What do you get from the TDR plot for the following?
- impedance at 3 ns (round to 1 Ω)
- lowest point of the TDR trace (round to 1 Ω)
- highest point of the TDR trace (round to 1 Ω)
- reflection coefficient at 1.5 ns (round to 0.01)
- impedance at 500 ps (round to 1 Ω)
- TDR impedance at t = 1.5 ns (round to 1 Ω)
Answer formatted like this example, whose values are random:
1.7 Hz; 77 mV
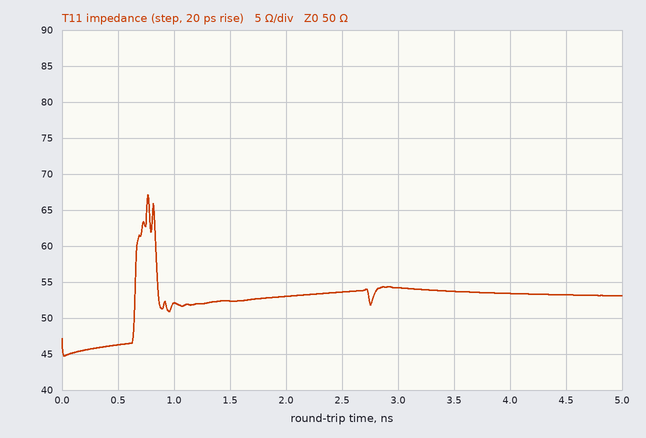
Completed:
54 Ω; 45 Ω; 67 Ω; +0.02; 46 Ω; 52 Ω
